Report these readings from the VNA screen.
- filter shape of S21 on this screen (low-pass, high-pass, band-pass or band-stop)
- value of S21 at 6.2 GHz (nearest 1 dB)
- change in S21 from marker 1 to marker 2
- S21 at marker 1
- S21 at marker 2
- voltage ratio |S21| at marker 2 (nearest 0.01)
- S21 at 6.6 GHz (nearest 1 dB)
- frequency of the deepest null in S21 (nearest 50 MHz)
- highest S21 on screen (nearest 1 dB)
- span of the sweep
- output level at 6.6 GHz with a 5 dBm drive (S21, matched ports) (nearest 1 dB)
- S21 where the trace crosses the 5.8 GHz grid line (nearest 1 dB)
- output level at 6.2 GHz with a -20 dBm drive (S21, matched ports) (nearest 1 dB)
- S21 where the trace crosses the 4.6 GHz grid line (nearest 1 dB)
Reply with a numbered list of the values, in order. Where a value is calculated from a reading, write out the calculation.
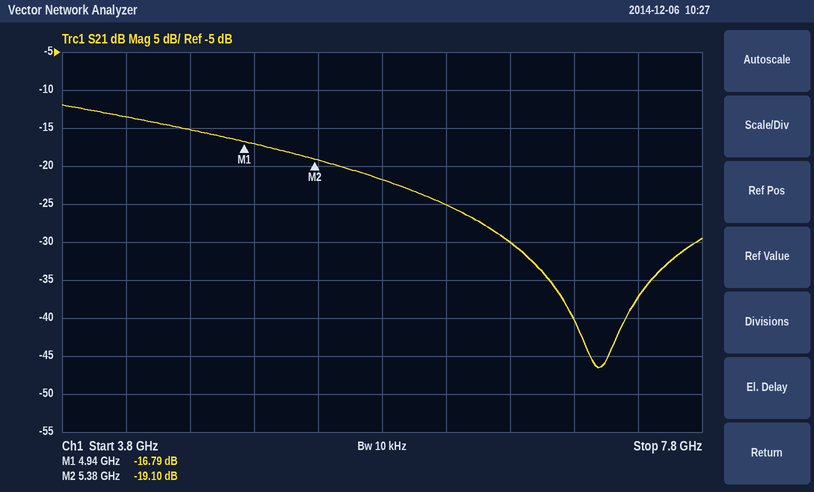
1. low-pass
2. -25 dB
3. -19.1 − (-16.79) = -2.31 dB
4. -16.79 dB
5. -19.10 dB
6. 10^(-19.1/20) ≈ 0.11
7. -30 dB
8. 7.15 GHz
9. -12 dB
10. 4 GHz
11. 5 dBm + (-30 dB) = -25 dBm
12. -22 dB
13. -20 dBm + (-25 dB) = -45 dBm
14. -15 dB
